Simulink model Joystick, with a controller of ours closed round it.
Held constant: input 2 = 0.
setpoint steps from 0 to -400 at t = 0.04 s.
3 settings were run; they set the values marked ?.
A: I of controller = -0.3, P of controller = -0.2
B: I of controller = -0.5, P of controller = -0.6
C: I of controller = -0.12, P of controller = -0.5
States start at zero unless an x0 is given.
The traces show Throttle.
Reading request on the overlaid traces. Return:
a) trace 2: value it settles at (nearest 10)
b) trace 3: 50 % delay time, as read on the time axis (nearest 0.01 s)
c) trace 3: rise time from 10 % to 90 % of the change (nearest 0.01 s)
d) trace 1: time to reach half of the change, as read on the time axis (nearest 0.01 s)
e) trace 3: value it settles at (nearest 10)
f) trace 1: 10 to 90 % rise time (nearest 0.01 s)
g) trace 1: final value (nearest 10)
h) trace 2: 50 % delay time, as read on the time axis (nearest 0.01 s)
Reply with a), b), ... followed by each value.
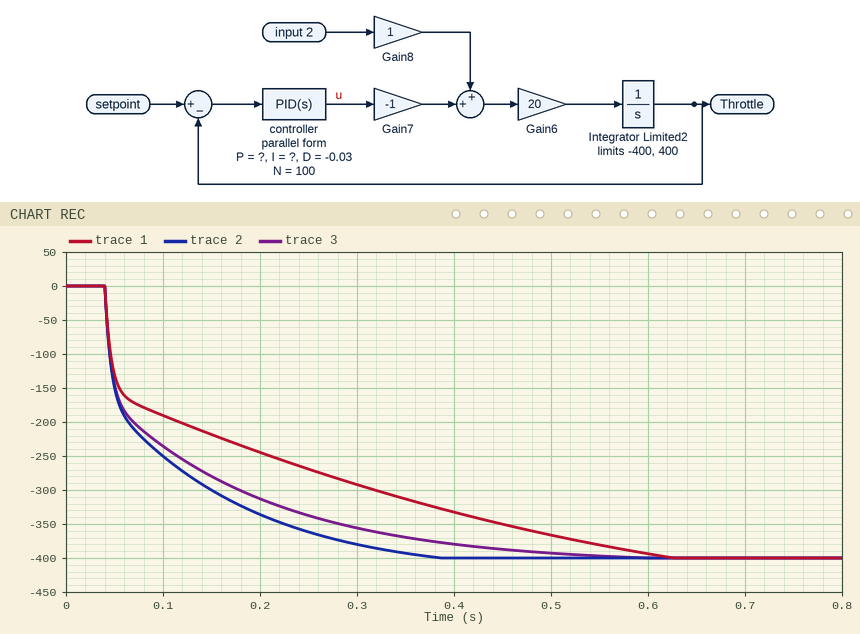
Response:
a) -400
b) 0.07 s
c) 0.27 s
d) 0.12 s
e) -400
f) 0.44 s
g) -400
h) 0.06 s
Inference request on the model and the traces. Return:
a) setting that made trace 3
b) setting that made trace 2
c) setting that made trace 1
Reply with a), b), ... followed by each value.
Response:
a) C
b) B
c) A
